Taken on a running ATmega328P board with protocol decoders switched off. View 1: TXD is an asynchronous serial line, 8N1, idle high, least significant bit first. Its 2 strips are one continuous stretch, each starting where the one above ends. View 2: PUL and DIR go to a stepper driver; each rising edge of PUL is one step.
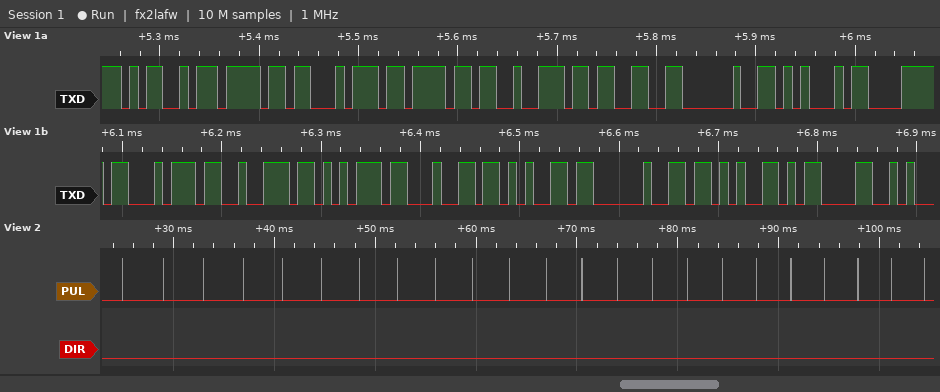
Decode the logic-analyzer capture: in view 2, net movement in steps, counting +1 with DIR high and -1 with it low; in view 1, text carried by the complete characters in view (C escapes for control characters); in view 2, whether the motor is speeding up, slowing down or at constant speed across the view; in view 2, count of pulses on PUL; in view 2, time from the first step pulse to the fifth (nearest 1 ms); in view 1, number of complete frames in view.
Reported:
-23
"Motor3 Extrude +\r"
speeding up
23
16 ms
17
